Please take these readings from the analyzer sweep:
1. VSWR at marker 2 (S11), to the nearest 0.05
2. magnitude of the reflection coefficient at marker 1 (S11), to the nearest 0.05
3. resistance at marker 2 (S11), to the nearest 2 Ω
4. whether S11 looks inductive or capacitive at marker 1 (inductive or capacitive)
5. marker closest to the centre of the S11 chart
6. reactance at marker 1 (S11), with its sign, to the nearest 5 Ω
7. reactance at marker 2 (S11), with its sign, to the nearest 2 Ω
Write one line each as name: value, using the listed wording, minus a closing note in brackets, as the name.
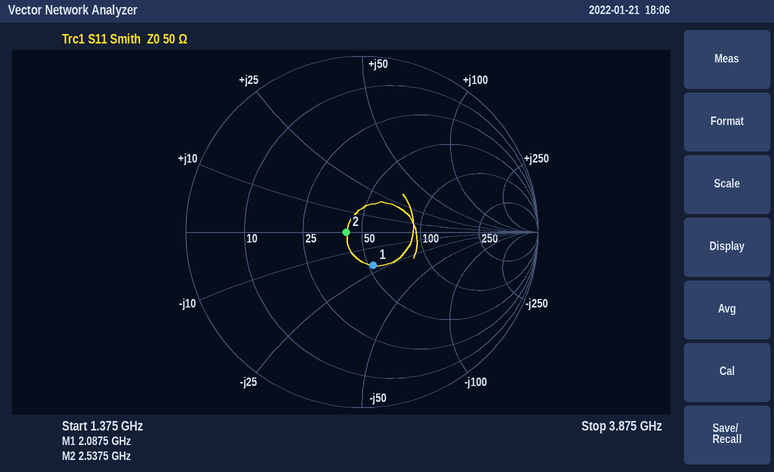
VSWR at marker 2 (S11), to the nearest 0.05: 1.20
magnitude of the reflection coefficient at marker 1 (S11), to the nearest 0.05: 0.20
resistance at marker 2 (S11), to the nearest 2 Ω: 42 Ω
whether S11 looks inductive or capacitive at marker 1: capacitive
marker closest to the centre of the S11 chart: marker 2
reactance at marker 1 (S11), with its sign, to the nearest 5 Ω: -20 Ω
reactance at marker 2 (S11), with its sign, to the nearest 2 Ω: 0 Ω
